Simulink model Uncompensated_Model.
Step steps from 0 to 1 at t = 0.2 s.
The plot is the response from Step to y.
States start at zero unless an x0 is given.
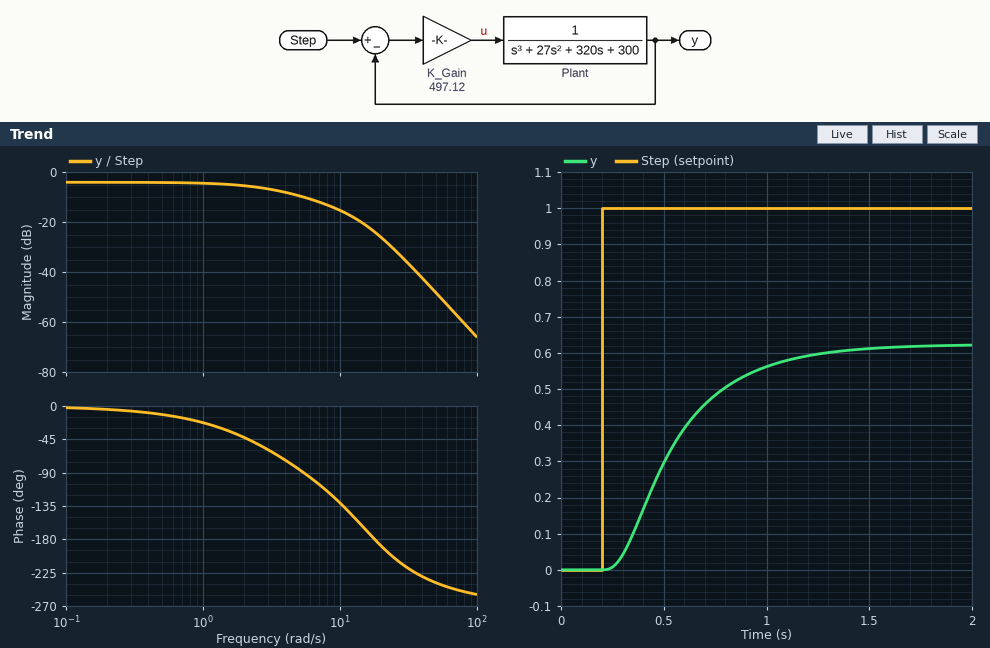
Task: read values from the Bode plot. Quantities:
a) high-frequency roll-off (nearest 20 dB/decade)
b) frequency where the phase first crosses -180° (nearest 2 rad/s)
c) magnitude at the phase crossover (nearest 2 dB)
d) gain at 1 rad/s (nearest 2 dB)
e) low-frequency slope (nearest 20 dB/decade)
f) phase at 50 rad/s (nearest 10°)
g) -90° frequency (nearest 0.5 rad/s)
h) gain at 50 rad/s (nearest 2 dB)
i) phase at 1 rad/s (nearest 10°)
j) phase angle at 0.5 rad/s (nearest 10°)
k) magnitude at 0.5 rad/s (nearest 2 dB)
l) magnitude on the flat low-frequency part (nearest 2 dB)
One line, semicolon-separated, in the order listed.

-60 dB/decade; 18 rad/s; -24 dB; -4 dB; 0 dB/decade; -240°; 5.5 rad/s; -48 dB; -20°; -10°; -4 dB; -4 dB
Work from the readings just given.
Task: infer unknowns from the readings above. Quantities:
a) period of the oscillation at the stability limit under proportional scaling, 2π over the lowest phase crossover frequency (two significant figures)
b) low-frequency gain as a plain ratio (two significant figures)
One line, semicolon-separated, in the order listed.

0.35 s; 0.63
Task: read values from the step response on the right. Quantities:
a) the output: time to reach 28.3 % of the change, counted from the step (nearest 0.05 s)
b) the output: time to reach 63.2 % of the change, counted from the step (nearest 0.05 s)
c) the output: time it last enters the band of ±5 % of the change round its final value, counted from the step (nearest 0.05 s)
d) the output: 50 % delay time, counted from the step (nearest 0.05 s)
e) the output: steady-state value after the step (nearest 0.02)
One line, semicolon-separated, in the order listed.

0.20 s; 0.40 s; 1.00 s; 0.30 s; 0.62
